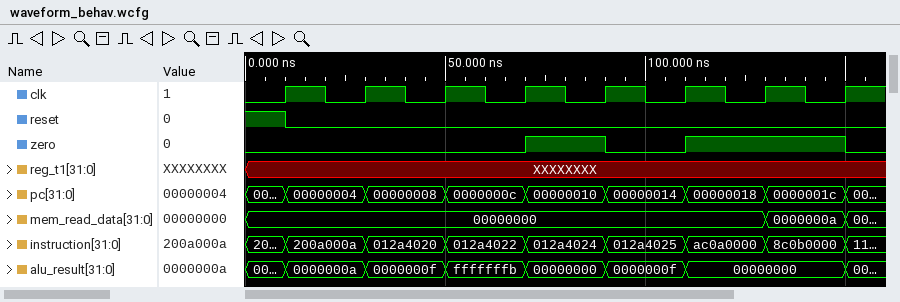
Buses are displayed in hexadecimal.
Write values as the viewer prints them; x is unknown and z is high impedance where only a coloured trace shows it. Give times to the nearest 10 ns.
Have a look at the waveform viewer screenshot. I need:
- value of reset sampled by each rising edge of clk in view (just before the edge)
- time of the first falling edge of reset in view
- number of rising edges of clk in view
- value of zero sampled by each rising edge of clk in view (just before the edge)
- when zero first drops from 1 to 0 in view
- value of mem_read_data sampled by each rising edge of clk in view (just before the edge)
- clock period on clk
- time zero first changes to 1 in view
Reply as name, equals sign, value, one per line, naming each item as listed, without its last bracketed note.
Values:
value of reset sampled by each rising edge of clk in view = 1 0 0 0 0 0 0 0
time of the first falling edge of reset in view = 10 ns
number of rising edges of clk in view = 8
value of zero sampled by each rising edge of clk in view = 0 0 0 0 1 0 1 1
when zero first drops from 1 to 0 in view = 90 ns
value of mem_read_data sampled by each rising edge of clk in view = 00000000, 00000000, 00000000, 00000000, 00000000, 00000000, 00000000, 0000000a
clock period on clk = 20 ns
time zero first changes to 1 in view = 70 ns
